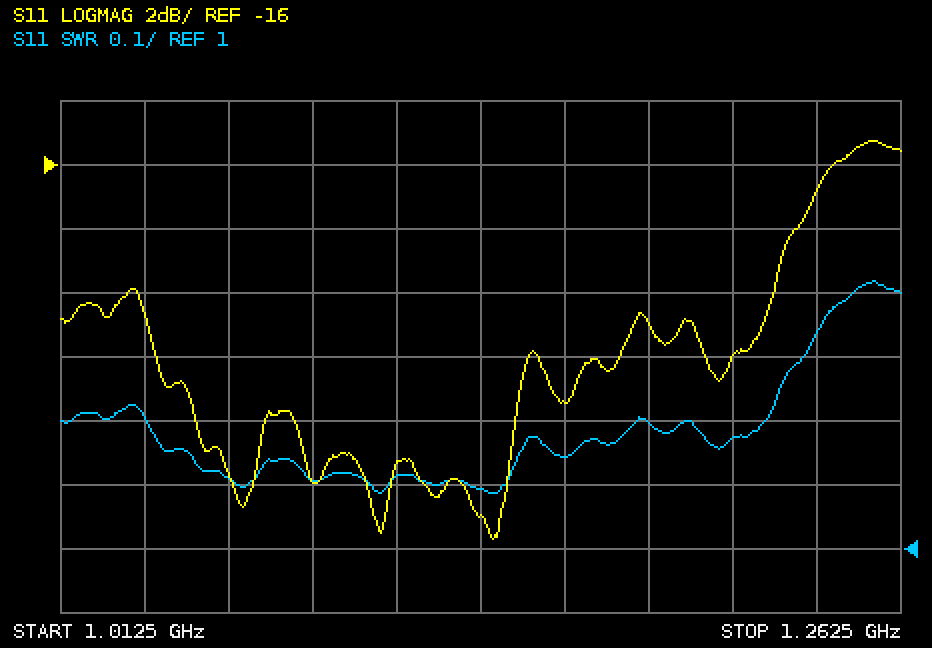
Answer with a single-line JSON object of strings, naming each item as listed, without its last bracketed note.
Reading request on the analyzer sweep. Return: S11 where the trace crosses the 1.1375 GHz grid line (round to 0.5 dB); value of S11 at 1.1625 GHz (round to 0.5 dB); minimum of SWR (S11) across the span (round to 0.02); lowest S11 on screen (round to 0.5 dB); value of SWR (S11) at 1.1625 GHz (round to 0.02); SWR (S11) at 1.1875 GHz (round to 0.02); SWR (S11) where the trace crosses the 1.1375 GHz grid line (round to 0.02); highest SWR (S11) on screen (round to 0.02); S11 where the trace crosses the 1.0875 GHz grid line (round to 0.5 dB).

{"S11 where the trace crosses the 1.1375 GHz grid line": "-27.0 dB", "value of S11 at 1.1625 GHz": "-23.5 dB", "minimum of SWR (S11) across the span": "1.08", "lowest S11 on screen": "-27.5 dB", "value of SWR (S11) at 1.1625 GHz": "1.14", "SWR (S11) at 1.1875 GHz": "1.20", "SWR (S11) where the trace crosses the 1.1375 GHz grid line": "1.10", "highest SWR (S11) on screen": "1.42", "S11 where the trace crosses the 1.0875 GHz grid line": "-26.0 dB"}
